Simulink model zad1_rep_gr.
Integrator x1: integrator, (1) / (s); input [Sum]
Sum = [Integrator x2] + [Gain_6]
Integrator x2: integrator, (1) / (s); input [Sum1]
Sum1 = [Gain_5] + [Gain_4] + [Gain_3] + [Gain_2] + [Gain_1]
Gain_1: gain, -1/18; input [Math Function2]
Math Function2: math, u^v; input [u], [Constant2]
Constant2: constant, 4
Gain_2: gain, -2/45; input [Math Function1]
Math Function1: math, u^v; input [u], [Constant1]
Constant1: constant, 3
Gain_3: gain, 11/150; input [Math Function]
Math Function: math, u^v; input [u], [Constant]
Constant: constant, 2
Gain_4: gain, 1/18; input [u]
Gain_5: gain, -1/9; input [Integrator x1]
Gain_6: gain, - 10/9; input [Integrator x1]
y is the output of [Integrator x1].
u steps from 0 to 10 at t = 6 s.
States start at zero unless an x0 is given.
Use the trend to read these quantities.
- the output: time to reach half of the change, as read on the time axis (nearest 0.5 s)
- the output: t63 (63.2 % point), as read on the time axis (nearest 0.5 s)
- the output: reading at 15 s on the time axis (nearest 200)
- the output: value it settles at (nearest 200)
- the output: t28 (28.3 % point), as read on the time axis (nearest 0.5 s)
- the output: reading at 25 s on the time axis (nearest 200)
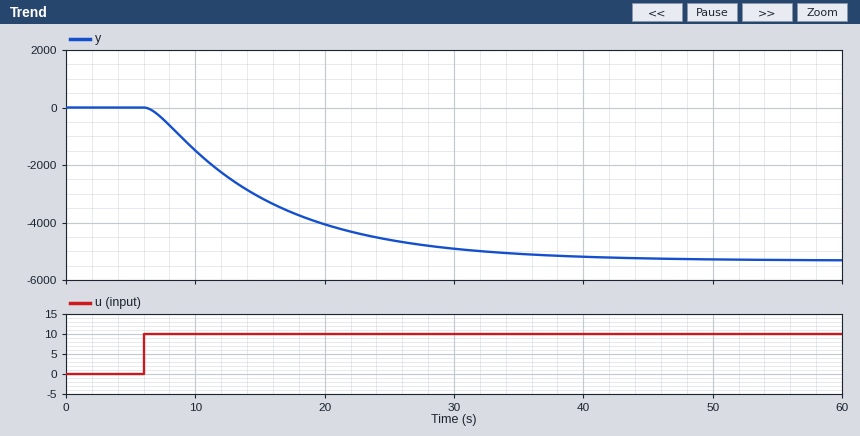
13.5 s
16.0 s
-3200
-5400
10.0 s
-4600
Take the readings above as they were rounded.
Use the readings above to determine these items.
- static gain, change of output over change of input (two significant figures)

-540
